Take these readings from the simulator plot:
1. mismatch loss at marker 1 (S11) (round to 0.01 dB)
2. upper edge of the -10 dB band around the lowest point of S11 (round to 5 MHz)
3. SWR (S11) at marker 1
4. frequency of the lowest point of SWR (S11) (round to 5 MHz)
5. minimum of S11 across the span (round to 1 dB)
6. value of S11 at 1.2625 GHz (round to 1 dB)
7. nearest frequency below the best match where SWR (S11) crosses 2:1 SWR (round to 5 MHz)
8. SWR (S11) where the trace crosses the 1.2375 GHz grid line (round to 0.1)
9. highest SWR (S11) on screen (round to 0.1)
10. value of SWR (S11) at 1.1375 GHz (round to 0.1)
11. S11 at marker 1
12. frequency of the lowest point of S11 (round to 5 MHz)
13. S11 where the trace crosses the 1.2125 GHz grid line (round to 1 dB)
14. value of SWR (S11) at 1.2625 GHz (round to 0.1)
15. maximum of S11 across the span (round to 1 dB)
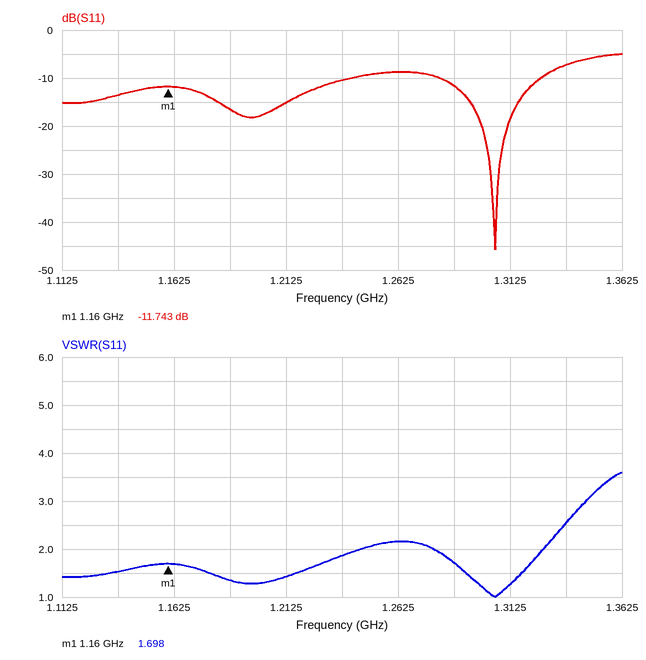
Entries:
0.30 dB
1.325 GHz
1.698
1.305 GHz
-46 dB
-9 dB
1.280 GHz
1.9
3.6
1.5
-11.743 dB
1.305 GHz
-15 dB
2.2
-5 dB
